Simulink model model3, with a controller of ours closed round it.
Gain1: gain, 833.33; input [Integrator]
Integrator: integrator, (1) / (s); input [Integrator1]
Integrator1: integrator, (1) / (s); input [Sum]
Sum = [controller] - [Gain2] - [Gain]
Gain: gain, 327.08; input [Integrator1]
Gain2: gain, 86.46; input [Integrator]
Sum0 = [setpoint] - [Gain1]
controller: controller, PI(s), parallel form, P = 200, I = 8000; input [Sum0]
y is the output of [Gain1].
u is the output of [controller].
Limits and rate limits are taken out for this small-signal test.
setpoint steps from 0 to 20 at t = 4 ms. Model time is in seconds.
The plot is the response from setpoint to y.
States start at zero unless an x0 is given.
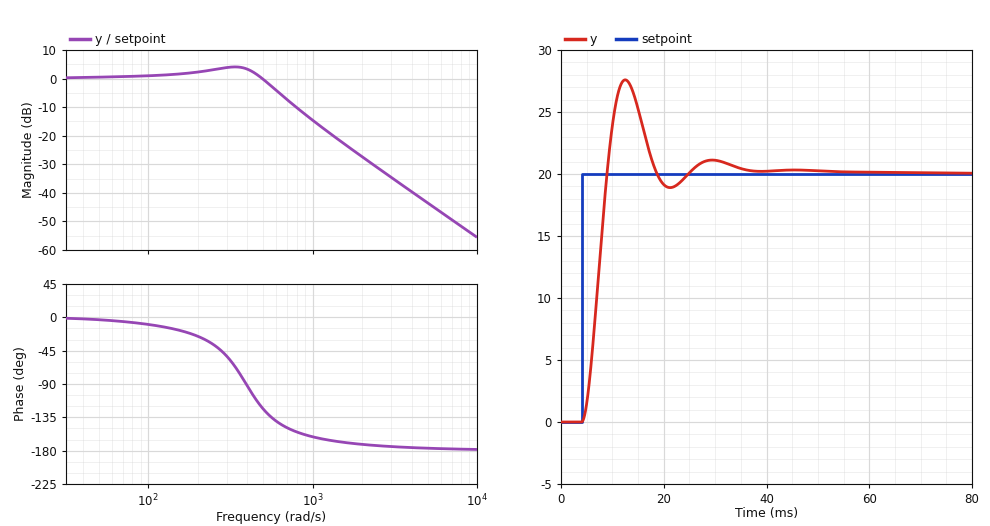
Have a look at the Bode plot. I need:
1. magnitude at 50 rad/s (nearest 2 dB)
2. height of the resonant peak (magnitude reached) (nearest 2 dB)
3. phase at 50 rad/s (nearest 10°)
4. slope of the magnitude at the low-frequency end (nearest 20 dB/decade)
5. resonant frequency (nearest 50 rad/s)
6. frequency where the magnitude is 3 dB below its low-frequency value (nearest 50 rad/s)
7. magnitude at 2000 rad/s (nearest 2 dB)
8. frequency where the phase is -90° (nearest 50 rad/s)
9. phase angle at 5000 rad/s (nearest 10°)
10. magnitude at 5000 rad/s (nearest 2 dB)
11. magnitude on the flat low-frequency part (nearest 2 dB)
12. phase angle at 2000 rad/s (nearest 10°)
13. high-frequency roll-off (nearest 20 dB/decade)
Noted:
0 dB
4 dB
0°
0 dB/decade
350 rad/s
550 rad/s
-28 dB
400 rad/s
-180°
-44 dB
0 dB
-170°
-40 dB/decade
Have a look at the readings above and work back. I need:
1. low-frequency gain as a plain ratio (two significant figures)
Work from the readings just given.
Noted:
1.0
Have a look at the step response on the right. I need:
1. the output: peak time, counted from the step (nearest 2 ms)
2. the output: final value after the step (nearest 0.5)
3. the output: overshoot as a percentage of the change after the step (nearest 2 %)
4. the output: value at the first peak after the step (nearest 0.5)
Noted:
8 ms
20.0
38 %
27.5
